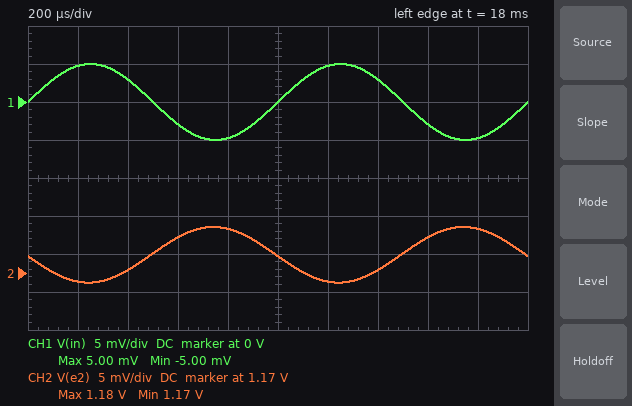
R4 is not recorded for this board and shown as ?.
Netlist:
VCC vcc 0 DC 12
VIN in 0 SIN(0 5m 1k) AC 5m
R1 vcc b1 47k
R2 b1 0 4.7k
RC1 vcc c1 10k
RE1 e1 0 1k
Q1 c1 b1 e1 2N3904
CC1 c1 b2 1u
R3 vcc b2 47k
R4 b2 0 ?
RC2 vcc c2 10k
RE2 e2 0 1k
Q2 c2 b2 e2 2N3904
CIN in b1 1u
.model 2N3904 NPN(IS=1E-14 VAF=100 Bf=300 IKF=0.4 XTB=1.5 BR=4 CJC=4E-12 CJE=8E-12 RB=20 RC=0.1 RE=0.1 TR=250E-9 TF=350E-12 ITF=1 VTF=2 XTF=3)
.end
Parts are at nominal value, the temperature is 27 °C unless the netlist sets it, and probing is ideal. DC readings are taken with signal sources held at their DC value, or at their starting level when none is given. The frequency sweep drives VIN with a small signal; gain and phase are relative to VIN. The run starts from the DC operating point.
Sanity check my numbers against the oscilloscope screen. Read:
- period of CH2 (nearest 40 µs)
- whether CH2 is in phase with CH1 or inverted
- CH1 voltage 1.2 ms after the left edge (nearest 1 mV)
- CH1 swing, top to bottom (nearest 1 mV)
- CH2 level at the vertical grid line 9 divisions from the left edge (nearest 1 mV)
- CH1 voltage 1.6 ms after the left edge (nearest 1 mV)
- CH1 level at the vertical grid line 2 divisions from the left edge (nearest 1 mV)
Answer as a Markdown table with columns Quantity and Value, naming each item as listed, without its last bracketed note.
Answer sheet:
| Quantity | Value |
|---|---|
| period of CH2 | 1.00 ms |
| whether CH2 is in phase with CH1 or inverted | inverted |
| CH1 voltage 1.2 ms after the left edge | 5 mV |
| CH1 swing, top to bottom | 10 mV |
| CH2 level at the vertical grid line 9 divisions from the left edge | 1.176 V |
| CH1 voltage 1.6 ms after the left edge | -3 mV |
| CH1 level at the vertical grid line 2 divisions from the left edge | 3 mV |
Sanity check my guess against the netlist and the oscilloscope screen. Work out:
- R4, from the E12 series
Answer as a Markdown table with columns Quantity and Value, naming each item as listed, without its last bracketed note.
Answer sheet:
| Quantity | Value |
|---|---|
| R4, from the E12 series | 15 kΩ |
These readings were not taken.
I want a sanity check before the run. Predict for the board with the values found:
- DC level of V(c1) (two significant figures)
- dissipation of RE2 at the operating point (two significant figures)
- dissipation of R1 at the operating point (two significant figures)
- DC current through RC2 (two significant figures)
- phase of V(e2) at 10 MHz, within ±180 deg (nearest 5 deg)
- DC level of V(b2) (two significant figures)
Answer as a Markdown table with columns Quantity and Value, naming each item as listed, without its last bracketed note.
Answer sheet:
| Quantity | Value |
|---|---|
| DC level of V(c1) | 7.5 V |
| dissipation of RE2 at the operating point | 1.4 mW |
| dissipation of R1 at the operating point | 2.5 mW |
| DC current through RC2 | 1.1 mA |
| phase of V(e2) at 10 MHz, within ±180 deg | 165 deg |
| DC level of V(b2) | 1.8 V |
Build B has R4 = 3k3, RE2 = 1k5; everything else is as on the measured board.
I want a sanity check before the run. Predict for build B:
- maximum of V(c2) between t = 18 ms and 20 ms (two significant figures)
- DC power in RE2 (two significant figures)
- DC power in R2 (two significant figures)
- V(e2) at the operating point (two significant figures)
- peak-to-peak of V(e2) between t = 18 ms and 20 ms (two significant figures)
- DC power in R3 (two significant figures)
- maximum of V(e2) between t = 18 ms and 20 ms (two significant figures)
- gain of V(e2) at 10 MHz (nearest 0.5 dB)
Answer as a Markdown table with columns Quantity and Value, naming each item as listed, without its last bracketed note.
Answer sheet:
| Quantity | Value |
|---|---|
| maximum of V(c2) between t = 18 ms and 20 ms | 11 V |
| DC power in RE2 | 23 µW |
| DC power in R2 | 250 µW |
| V(e2) at the operating point | 190 mV |
| peak-to-peak of V(e2) between t = 18 ms and 20 ms | 19 mV |
| DC power in R3 | 2.7 mW |
| maximum of V(e2) between t = 18 ms and 20 ms | 200 mV |
| gain of V(e2) at 10 MHz | -1.5 dB |
